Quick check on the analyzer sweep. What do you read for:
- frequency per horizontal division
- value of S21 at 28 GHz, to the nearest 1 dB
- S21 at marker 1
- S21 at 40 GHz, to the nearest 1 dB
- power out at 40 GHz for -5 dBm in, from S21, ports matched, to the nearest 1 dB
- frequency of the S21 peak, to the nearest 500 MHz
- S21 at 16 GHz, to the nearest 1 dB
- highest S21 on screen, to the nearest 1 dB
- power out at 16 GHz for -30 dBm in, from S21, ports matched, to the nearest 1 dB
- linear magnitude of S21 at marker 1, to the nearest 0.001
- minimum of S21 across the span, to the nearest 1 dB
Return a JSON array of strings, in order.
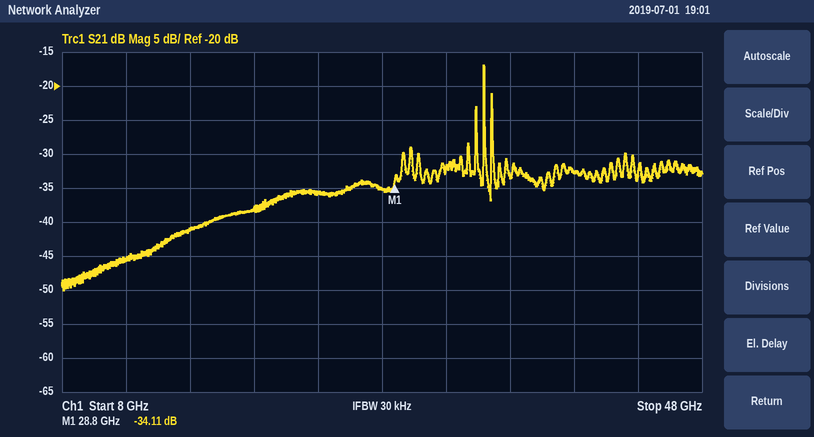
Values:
["4 GHz", "-35 dB", "-34.11 dB", "-33 dB", "-38 dBm", "34.5 GHz", "-41 dB", "-17 dB", "-71 dBm", "0.020", "-50 dB"]
